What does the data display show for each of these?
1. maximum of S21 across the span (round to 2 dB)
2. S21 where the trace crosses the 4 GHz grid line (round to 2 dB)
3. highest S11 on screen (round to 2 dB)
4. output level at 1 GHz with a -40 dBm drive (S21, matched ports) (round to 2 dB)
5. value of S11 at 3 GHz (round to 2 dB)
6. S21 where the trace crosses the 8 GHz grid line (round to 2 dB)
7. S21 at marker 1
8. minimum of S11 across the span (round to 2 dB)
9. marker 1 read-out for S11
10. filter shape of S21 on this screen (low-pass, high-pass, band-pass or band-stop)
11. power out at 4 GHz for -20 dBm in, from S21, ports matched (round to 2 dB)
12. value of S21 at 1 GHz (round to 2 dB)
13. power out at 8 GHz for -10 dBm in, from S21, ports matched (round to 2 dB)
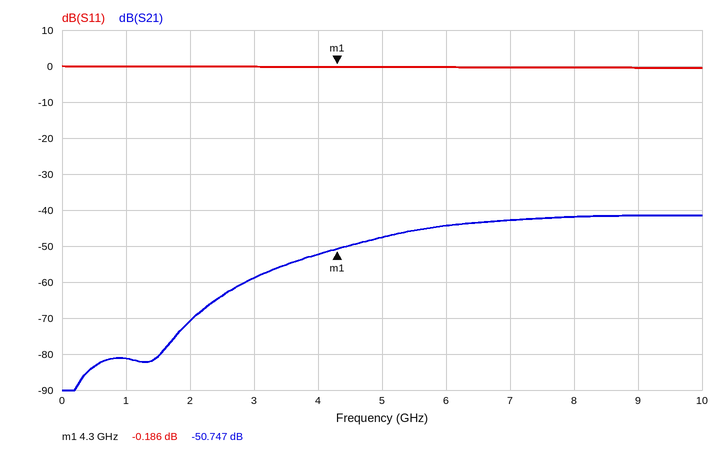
-42 dB
-52 dB
0 dB
-122 dBm
0 dB
-42 dB
-50.747 dB
0 dB
-0.186 dB
high-pass
-72 dBm
-82 dB
-52 dBm
